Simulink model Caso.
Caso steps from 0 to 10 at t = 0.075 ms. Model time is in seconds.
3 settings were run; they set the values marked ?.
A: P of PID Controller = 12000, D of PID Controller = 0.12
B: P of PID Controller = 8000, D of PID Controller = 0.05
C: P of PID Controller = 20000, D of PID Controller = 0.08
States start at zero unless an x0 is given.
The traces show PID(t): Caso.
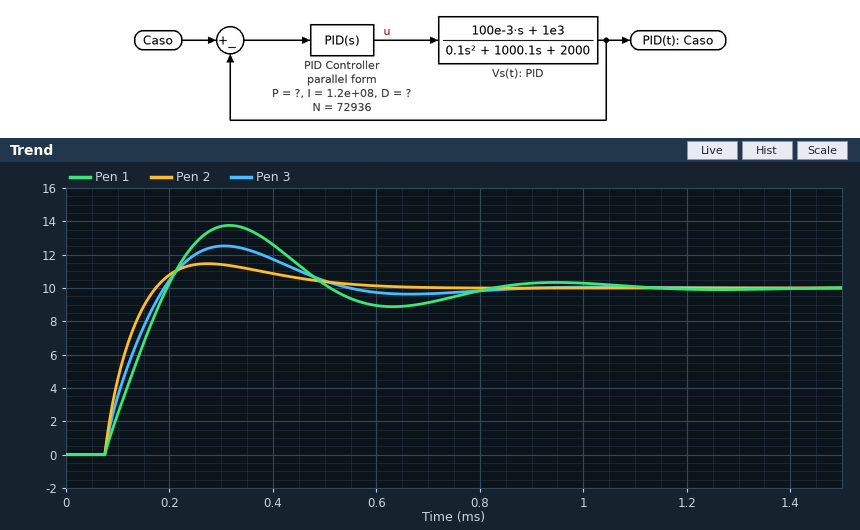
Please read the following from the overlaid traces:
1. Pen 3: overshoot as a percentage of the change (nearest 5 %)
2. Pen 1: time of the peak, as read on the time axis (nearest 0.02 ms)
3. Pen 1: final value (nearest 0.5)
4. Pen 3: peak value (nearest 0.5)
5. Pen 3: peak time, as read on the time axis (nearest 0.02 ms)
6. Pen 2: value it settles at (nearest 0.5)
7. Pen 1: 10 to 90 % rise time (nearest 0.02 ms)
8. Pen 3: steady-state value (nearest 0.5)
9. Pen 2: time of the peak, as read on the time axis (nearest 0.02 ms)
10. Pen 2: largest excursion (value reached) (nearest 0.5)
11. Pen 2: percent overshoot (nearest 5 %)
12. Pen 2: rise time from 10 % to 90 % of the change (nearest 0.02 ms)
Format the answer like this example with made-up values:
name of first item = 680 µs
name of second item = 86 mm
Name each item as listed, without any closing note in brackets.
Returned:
Pen 3: overshoot as a percentage of the change = 25 %
Pen 1: time of the peak, as read on the time axis = 0.32 ms
Pen 1: final value = 10.0
Pen 3: peak value = 12.5
Pen 3: peak time, as read on the time axis = 0.30 ms
Pen 2: value it settles at = 10.0
Pen 1: 10 to 90 % rise time = 0.10 ms
Pen 3: steady-state value = 10.0
Pen 2: time of the peak, as read on the time axis = 0.28 ms
Pen 2: largest excursion (value reached) = 11.5
Pen 2: percent overshoot = 15 %
Pen 2: rise time from 10 % to 90 % of the change = 0.08 ms
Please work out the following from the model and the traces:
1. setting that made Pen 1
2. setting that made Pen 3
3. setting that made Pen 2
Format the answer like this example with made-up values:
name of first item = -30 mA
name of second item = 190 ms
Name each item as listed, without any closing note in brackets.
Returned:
setting that made Pen 1 = B
setting that made Pen 3 = A
setting that made Pen 2 = C
